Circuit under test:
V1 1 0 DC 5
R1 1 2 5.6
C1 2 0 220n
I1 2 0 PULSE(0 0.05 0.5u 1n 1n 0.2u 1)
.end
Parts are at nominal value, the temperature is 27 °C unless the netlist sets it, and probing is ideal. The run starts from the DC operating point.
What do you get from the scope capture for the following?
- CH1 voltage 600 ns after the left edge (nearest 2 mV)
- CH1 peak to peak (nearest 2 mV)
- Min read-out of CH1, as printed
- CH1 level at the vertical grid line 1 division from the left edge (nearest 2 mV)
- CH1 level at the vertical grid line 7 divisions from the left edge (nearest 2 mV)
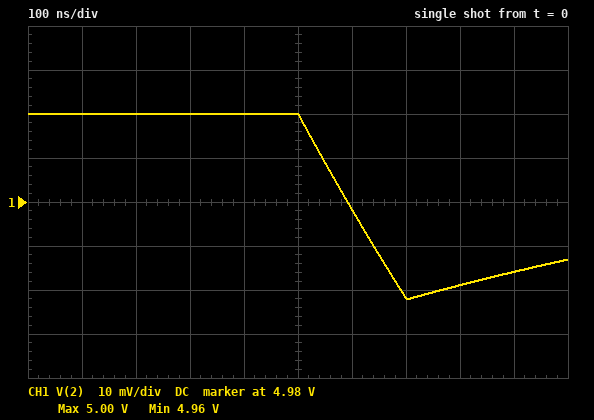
4.978 V
42 mV
4.96 V
5.000 V
4.958 V
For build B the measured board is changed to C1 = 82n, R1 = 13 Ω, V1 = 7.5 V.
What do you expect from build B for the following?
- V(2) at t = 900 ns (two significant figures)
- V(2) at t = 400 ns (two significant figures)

7.4 V
7.5 V
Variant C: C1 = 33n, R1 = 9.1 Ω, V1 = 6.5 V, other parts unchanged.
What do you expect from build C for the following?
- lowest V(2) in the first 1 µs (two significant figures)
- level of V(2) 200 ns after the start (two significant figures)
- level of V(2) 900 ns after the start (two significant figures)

6.3 V
6.5 V
6.4 V
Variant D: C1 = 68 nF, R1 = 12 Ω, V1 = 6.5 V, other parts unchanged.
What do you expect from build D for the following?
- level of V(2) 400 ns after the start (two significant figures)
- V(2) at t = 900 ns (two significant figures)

6.5 V
6.4 V
